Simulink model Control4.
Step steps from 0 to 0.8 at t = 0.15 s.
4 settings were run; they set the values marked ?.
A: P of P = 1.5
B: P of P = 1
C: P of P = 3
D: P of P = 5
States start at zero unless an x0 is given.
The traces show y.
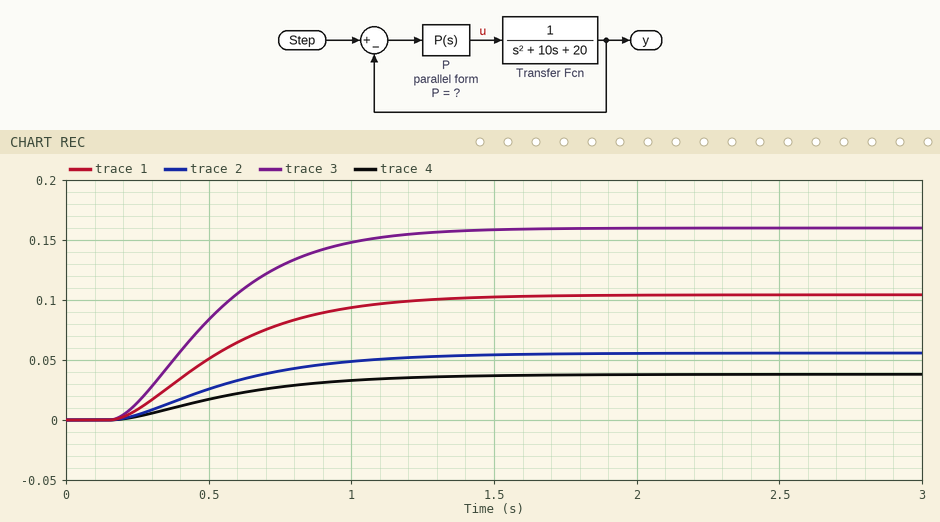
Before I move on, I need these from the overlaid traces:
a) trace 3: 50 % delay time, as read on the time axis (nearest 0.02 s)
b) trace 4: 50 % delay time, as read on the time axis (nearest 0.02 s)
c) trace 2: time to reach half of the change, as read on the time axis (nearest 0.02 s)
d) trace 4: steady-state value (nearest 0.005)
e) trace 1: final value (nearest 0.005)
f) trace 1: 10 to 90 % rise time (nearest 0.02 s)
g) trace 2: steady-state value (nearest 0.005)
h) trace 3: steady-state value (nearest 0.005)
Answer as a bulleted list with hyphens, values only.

- 0.48 s
- 0.54 s
- 0.52 s
- 0.040
- 0.105
- 0.74 s
- 0.055
- 0.160
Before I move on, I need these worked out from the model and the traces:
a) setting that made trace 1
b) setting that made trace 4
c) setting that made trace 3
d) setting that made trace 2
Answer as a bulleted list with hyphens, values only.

- C
- B
- D
- A
